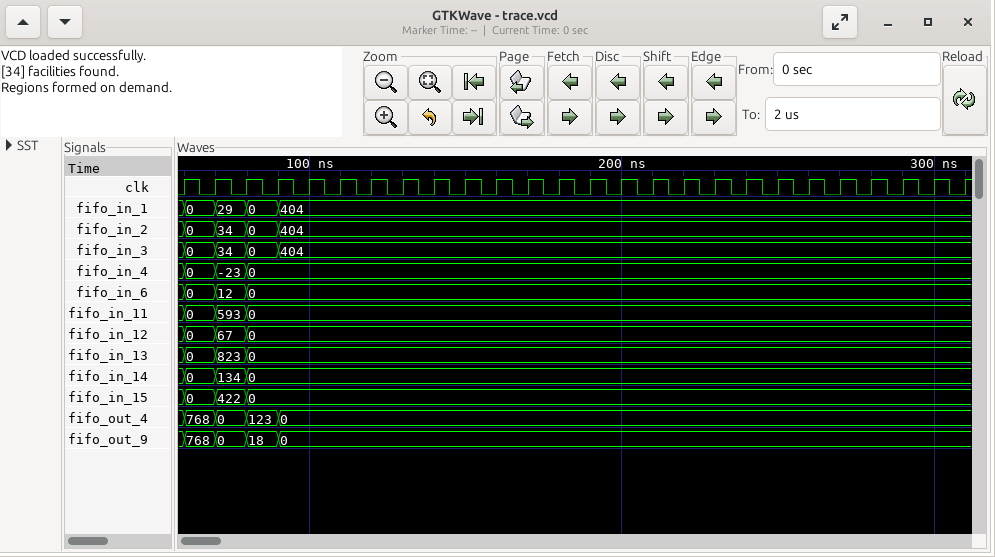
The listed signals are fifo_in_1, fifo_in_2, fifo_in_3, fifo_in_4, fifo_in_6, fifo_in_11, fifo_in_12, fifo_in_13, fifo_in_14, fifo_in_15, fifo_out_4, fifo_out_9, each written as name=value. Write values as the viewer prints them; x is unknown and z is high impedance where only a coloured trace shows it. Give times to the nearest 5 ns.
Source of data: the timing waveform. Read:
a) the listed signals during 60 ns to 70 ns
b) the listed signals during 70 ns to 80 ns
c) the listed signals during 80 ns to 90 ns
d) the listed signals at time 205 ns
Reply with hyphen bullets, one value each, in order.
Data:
- fifo_in_1=0, fifo_in_2=0, fifo_in_3=0, fifo_in_4=0, fifo_in_6=0, fifo_in_11=0, fifo_in_12=0, fifo_in_13=0, fifo_in_14=0, fifo_in_15=0, fifo_out_4=768, fifo_out_9=768
- fifo_in_1=29, fifo_in_2=34, fifo_in_3=34, fifo_in_4=-23, fifo_in_6=12, fifo_in_11=593, fifo_in_12=67, fifo_in_13=823, fifo_in_14=134, fifo_in_15=422, fifo_out_4=0, fifo_out_9=0
- fifo_in_1=0, fifo_in_2=0, fifo_in_3=0, fifo_in_4=0, fifo_in_6=0, fifo_in_11=0, fifo_in_12=0, fifo_in_13=0, fifo_in_14=0, fifo_in_15=0, fifo_out_4=123, fifo_out_9=18
- fifo_in_1=404, fifo_in_2=404, fifo_in_3=404, fifo_in_4=0, fifo_in_6=0, fifo_in_11=0, fifo_in_12=0, fifo_in_13=0, fifo_in_14=0, fifo_in_15=0, fifo_out_4=0, fifo_out_9=0
